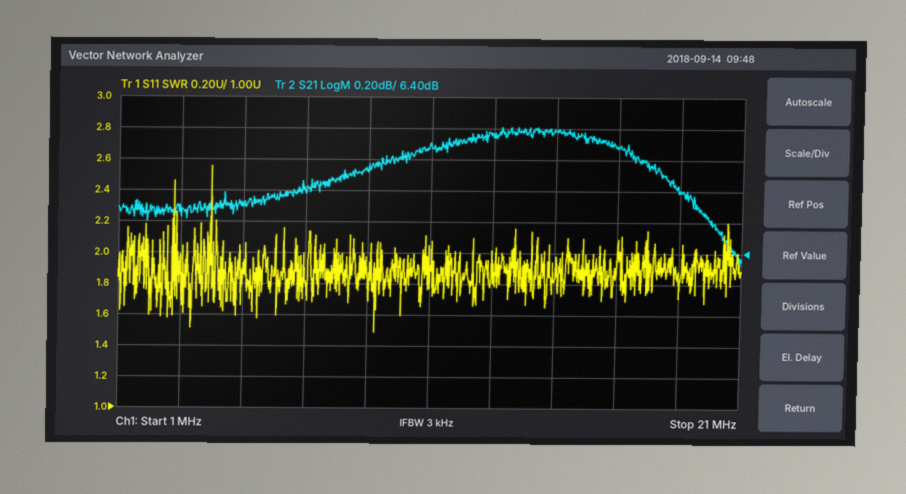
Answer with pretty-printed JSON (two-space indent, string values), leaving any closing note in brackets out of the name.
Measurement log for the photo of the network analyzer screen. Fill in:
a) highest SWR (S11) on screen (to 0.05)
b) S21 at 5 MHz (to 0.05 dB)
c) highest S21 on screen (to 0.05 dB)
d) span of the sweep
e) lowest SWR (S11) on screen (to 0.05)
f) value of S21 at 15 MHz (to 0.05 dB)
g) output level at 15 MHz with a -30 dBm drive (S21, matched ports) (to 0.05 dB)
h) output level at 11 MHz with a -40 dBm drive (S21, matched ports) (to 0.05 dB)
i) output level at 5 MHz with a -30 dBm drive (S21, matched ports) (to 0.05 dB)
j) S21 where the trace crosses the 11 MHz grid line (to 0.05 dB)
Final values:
{
  "highest SWR (S11) on screen": "2.55",
  "S21 at 5 MHz": "6.70 dB",
  "highest S21 on screen": "7.20 dB",
  "span of the sweep": "20 MHz",
  "lowest SWR (S11) on screen": "1.50",
  "value of S21 at 15 MHz": "7.20 dB",
  "output level at 15 MHz with a -30 dBm drive (S21, matched ports)": "-22.80 dBm",
  "output level at 11 MHz with a -40 dBm drive (S21, matched ports)": "-32.90 dBm",
  "output level at 5 MHz with a -30 dBm drive (S21, matched ports)": "-23.30 dBm",
  "S21 where the trace crosses the 11 MHz grid line": "7.10 dB"
}
